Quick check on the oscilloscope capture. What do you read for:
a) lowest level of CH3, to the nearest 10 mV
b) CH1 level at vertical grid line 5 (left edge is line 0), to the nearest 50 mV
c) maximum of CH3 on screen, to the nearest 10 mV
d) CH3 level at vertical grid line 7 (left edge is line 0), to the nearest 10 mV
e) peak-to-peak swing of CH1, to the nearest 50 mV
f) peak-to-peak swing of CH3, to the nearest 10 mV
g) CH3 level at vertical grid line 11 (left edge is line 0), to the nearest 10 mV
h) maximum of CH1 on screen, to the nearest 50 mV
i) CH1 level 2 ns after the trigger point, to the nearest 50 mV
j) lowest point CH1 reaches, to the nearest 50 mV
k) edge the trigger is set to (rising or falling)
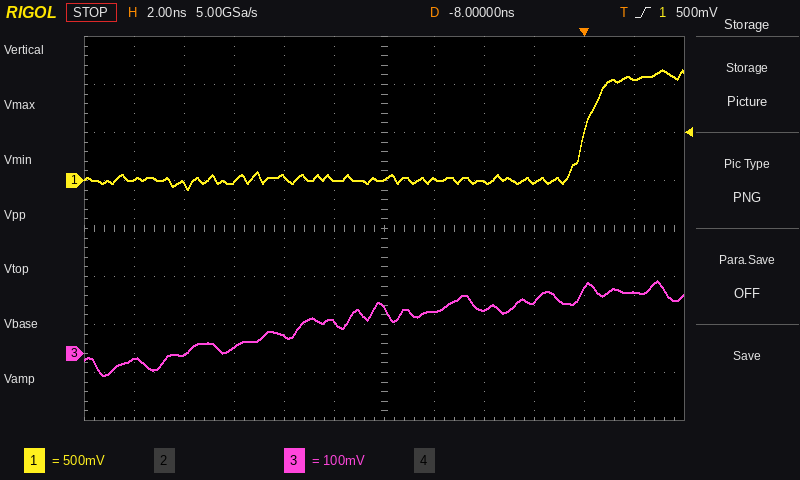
-50 mV
0 mV
150 mV
90 mV
1.25 V
200 mV
130 mV
1.15 V
1.05 V
-100 mV
rising
